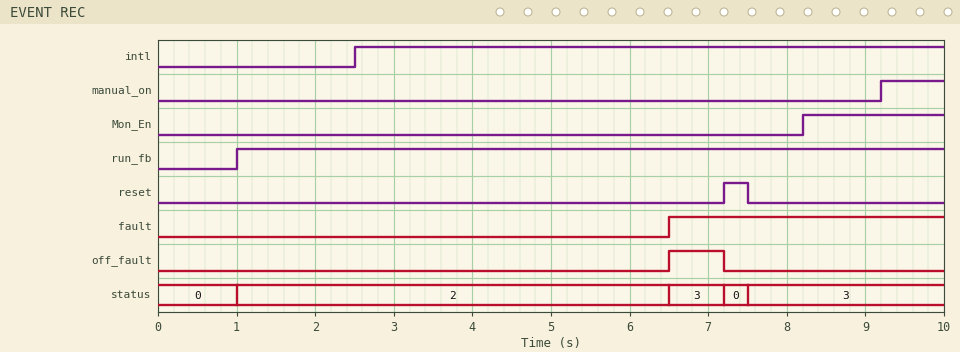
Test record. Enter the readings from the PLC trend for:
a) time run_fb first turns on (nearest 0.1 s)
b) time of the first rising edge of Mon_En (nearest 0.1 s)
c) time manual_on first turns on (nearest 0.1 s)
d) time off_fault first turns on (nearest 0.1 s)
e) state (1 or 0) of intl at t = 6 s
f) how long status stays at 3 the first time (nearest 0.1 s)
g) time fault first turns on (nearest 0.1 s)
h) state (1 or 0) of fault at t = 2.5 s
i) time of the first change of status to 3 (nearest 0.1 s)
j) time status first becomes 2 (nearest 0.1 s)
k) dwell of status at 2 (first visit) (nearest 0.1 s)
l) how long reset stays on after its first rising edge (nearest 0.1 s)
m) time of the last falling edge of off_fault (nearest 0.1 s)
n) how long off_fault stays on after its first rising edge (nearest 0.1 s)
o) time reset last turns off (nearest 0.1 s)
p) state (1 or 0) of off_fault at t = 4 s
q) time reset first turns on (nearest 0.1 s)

1.0 s
8.2 s
9.2 s
6.5 s
1
0.7 s
6.5 s
0
6.5 s
1.0 s
5.5 s
0.3 s
7.2 s
0.7 s
7.5 s
0
7.2 s
